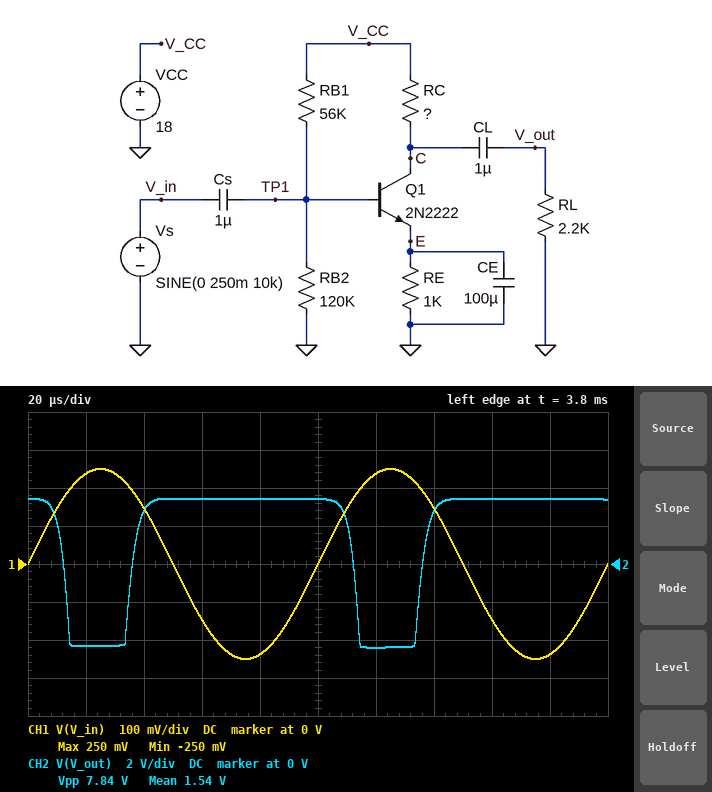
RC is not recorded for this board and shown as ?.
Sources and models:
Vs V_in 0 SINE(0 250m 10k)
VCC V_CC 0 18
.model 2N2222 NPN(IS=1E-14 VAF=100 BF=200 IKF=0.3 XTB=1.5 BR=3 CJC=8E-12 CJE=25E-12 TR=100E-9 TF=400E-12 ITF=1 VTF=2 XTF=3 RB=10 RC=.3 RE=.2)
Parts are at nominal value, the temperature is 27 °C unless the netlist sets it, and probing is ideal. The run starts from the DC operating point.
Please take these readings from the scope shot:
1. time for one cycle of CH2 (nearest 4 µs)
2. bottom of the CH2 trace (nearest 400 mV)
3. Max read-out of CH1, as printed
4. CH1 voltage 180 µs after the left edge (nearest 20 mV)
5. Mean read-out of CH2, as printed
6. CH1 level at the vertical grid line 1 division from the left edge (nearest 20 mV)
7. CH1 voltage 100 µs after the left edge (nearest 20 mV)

100 µs
-4.4 V
250 mV
-240 mV
1.54 V
240 mV
0 V
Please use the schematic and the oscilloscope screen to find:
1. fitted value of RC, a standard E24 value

4.3 kΩ
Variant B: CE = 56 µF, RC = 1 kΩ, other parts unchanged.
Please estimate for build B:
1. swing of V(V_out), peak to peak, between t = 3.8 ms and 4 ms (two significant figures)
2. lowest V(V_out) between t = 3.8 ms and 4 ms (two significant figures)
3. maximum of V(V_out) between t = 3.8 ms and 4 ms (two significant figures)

8.1 V
-5.1 V
3.0 V
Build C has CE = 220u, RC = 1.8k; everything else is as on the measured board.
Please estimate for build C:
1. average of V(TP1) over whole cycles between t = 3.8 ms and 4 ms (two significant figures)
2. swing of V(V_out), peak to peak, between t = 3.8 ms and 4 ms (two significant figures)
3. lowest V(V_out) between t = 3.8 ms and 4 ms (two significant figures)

6.9 V
8.8 V
-5.3 V
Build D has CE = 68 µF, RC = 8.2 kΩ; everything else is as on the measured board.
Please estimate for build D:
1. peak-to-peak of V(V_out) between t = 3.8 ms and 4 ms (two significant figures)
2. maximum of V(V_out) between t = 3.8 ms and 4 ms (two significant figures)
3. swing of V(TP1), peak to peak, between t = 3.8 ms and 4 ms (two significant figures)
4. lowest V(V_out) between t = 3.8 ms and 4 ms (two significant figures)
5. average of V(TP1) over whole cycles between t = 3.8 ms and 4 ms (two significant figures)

5.8 V
2.7 V
500 mV
-3.1 V
2.6 V
